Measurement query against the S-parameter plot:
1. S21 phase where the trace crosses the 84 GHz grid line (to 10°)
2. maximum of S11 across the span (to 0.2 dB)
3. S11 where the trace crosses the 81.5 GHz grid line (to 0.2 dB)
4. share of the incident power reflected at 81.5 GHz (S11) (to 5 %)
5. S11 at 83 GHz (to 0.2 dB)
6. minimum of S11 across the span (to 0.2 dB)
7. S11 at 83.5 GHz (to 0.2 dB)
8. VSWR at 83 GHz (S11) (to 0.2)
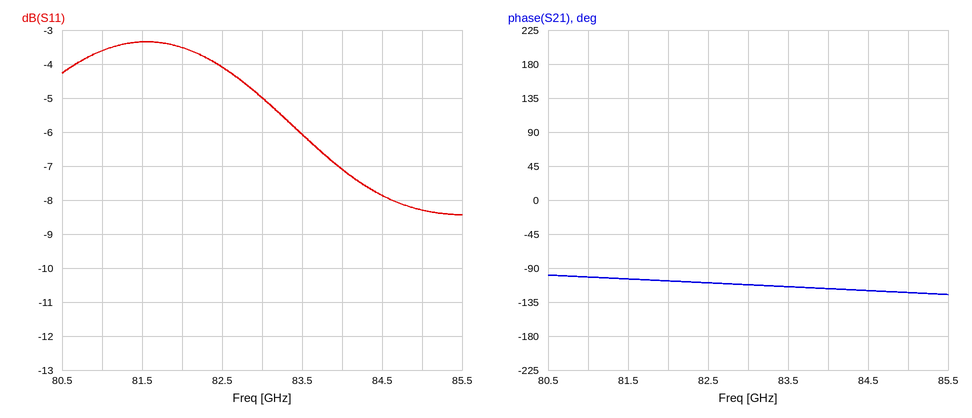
-120°
-3.4 dB
-3.4 dB
45 %
-5.0 dB
-8.4 dB
-6.0 dB
3.6
